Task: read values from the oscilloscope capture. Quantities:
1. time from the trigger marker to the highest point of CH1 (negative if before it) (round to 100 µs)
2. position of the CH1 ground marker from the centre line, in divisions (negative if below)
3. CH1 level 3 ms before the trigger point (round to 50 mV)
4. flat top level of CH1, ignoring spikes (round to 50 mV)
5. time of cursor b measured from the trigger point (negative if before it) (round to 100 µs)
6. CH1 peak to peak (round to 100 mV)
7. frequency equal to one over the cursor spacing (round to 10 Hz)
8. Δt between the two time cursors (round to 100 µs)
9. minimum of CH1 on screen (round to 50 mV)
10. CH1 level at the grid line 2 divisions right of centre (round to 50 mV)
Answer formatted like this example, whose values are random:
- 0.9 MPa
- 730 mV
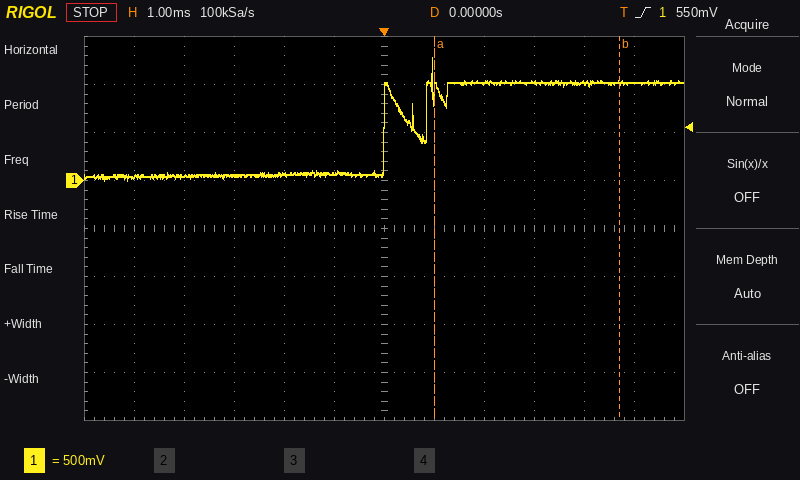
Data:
- +1.0 ms
- +1.0 div
- 50 mV
- 1.00 V
- +4.7 ms
- 1.30 V
- 270 Hz
- 3.7 ms
- 0 mV
- 1.00 V
